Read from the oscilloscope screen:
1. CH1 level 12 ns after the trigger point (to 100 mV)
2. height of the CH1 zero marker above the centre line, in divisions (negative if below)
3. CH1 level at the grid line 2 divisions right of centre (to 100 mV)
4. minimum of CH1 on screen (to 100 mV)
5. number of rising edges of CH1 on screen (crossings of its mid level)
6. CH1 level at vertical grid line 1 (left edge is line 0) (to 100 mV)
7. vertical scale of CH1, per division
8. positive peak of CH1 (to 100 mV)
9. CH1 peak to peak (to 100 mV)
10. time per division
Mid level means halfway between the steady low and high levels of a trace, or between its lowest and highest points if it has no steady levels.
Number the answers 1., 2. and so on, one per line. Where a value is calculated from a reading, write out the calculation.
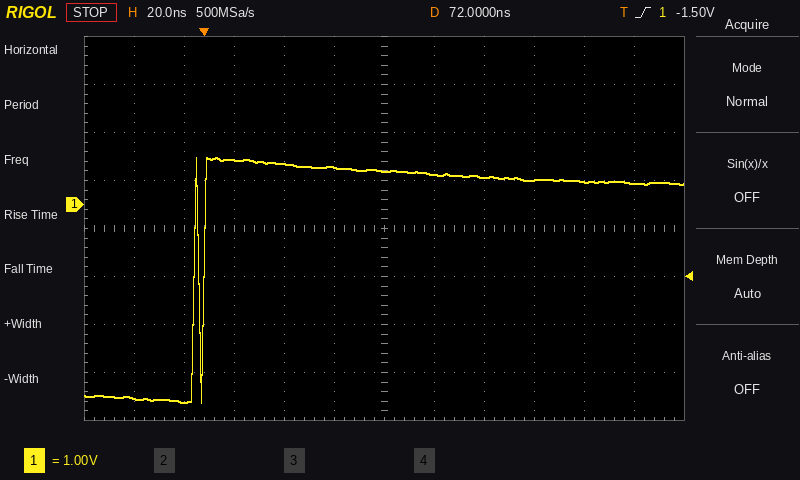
1. 900 mV
2. +0.5 div
3. 600 mV
4. -4.1 V
5. 2
6. -4.0 V
7. 1 V
8. 1.0 V
9. 1.0 V − (-4.1 V) = 5.1 V
10. 20 ns
